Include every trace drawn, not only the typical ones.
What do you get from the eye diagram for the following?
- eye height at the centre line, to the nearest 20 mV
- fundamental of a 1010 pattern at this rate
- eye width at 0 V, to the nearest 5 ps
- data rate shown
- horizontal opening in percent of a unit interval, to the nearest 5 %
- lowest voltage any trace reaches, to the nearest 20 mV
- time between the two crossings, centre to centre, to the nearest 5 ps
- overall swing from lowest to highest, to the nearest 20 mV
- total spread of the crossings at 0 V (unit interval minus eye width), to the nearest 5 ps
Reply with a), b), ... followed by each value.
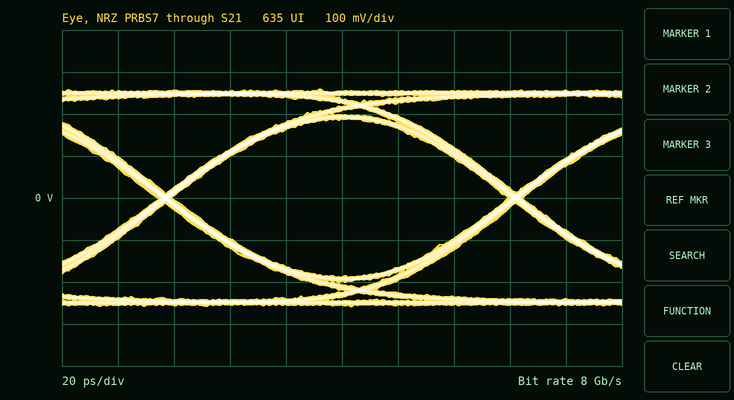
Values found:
a) 380 mV
b) 4 GHz
c) 120 ps
d) 8 Gb/s
e) 95 %
f) -260 mV
g) 125 ps
h) 520 mV
i) 5 ps
